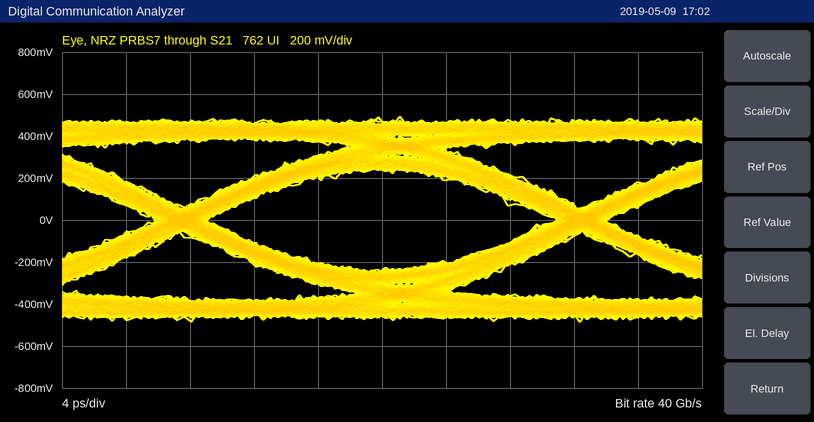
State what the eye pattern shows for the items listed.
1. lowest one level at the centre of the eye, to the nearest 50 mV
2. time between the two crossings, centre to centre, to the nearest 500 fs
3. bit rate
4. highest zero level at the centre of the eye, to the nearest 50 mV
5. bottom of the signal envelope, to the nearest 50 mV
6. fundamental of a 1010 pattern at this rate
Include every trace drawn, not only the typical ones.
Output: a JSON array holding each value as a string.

["250 mV", "25.0 ps", "40 Gb/s", "-250 mV", "-500 mV", "20 GHz"]
